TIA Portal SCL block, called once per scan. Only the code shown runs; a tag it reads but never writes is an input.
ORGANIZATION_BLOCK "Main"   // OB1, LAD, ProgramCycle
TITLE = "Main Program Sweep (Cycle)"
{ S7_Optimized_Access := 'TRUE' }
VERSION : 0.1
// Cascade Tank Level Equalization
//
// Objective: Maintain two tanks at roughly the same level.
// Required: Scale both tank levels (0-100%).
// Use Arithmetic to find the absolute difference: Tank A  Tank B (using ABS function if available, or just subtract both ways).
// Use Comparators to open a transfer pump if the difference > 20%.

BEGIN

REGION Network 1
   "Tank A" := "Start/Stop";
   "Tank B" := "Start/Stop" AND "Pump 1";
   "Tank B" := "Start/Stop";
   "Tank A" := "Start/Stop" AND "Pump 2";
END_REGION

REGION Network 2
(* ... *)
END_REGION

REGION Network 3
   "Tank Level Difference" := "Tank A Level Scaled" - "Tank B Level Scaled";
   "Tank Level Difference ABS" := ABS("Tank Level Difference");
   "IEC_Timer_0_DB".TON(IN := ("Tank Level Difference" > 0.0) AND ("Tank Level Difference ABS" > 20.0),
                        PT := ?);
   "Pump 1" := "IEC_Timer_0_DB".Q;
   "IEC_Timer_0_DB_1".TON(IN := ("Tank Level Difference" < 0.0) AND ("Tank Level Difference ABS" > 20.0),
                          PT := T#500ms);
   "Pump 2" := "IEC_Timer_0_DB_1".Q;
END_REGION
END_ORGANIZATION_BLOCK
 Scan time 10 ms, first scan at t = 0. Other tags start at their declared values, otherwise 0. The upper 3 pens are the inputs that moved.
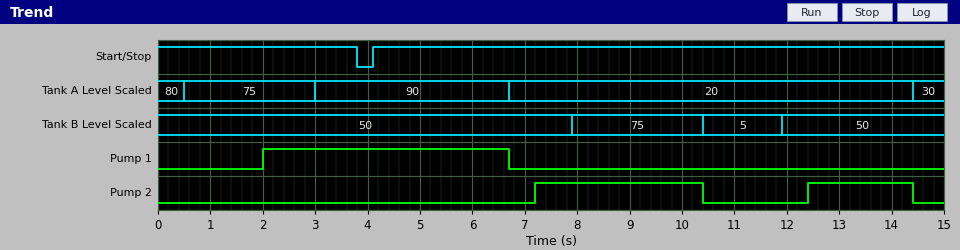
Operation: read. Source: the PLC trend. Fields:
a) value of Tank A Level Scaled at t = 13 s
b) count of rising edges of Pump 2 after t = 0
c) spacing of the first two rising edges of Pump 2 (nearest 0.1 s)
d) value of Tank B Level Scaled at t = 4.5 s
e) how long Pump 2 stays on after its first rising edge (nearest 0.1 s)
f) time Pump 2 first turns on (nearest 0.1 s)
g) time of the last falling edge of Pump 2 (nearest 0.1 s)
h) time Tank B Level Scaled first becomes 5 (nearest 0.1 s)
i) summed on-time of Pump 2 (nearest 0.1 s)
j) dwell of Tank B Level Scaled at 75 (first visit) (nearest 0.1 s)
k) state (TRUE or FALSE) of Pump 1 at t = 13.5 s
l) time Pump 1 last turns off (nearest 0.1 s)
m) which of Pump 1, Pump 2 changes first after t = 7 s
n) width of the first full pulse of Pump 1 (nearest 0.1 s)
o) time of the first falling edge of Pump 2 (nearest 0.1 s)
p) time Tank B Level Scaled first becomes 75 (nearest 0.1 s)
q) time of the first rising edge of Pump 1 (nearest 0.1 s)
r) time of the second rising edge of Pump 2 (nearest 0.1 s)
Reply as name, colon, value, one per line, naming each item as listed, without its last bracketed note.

value of Tank A Level Scaled at t = 13 s: 20
count of rising edges of Pump 2 after t = 0: 2
spacing of the first two rising edges of Pump 2: 5.2 s
value of Tank B Level Scaled at t = 4.5 s: 50
how long Pump 2 stays on after its first rising edge: 3.2 s
time Pump 2 first turns on: 7.2 s
time of the last falling edge of Pump 2: 14.4 s
time Tank B Level Scaled first becomes 5: 10.4 s
summed on-time of Pump 2: 5.2 s
dwell of Tank B Level Scaled at 75 (first visit): 2.5 s
state (TRUE or FALSE) of Pump 1 at t = 13.5 s: FALSE
time Pump 1 last turns off: 6.7 s
which of Pump 1, Pump 2 changes first after t = 7 s: Pump 2
width of the first full pulse of Pump 1: 4.7 s
time of the first falling edge of Pump 2: 10.4 s
time Tank B Level Scaled first becomes 75: 7.9 s
time of the first rising edge of Pump 1: 2.0 s
time of the second rising edge of Pump 2: 12.4 s
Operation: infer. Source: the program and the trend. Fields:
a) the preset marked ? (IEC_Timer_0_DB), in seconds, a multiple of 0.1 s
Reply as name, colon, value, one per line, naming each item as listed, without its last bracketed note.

the preset marked ? (IEC_Timer_0_DB), in seconds, a multiple of 0.1 s: 2.0 s
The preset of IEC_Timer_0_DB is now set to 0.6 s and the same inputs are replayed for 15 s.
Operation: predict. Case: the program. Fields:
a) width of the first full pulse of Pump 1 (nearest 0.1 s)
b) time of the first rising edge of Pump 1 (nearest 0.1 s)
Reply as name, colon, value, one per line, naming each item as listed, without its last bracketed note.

width of the first full pulse of Pump 1: 6.1 s
time of the first rising edge of Pump 1: 0.6 s
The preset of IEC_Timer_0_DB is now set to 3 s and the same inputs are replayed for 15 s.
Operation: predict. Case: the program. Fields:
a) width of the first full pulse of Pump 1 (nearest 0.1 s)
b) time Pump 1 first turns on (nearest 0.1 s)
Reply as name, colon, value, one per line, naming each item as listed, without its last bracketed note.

width of the first full pulse of Pump 1: 3.7 s
time Pump 1 first turns on: 3.0 s
